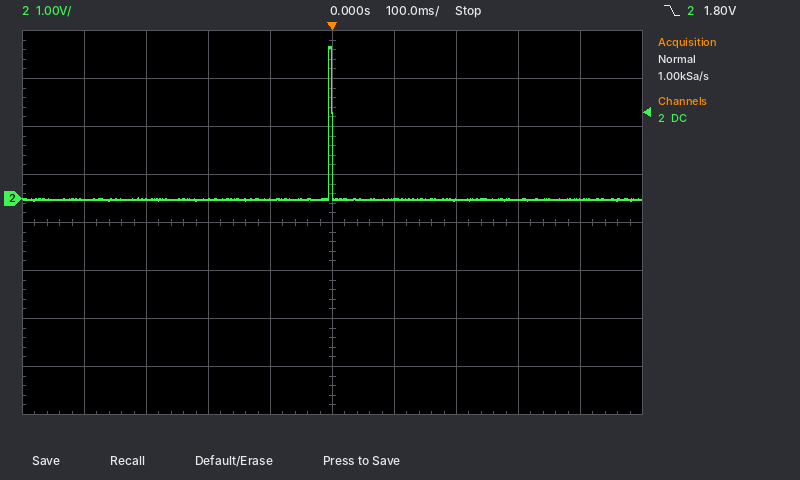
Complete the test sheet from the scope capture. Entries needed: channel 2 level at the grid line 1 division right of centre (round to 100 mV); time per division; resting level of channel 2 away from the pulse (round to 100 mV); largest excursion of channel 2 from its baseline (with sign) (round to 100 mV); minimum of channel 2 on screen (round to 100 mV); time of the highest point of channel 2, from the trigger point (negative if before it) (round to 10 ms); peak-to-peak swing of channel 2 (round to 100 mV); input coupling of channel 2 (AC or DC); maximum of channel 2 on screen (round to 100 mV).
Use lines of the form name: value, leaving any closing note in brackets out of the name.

channel 2 level at the grid line 1 division right of centre: 0.0 V
time per division: 100 ms
resting level of channel 2 away from the pulse: 0.0 V
largest excursion of channel 2 from its baseline (with sign): +3.2 V
minimum of channel 2 on screen: 0.0 V
time of the highest point of channel 2, from the trigger point (negative if before it): 0 ms
peak-to-peak swing of channel 2: 3.2 V
input coupling of channel 2: DC
maximum of channel 2 on screen: 3.2 V
